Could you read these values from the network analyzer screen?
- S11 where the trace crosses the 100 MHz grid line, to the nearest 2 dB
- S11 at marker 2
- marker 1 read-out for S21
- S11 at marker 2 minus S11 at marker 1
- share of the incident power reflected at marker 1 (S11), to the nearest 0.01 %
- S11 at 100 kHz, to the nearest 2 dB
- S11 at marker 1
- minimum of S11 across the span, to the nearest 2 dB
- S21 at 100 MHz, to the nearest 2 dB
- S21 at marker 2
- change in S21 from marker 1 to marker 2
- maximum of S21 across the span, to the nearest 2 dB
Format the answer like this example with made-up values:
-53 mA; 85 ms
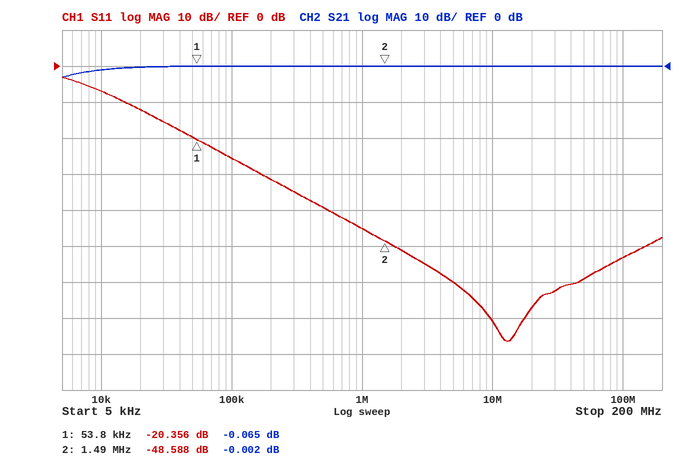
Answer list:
-54 dB; -48.588 dB; -0.065 dB; -28.232 dB; 0.92 %; -26 dB; -20.356 dB; -76 dB; 0 dB; -0.002 dB; 0.063 dB; 0 dB
